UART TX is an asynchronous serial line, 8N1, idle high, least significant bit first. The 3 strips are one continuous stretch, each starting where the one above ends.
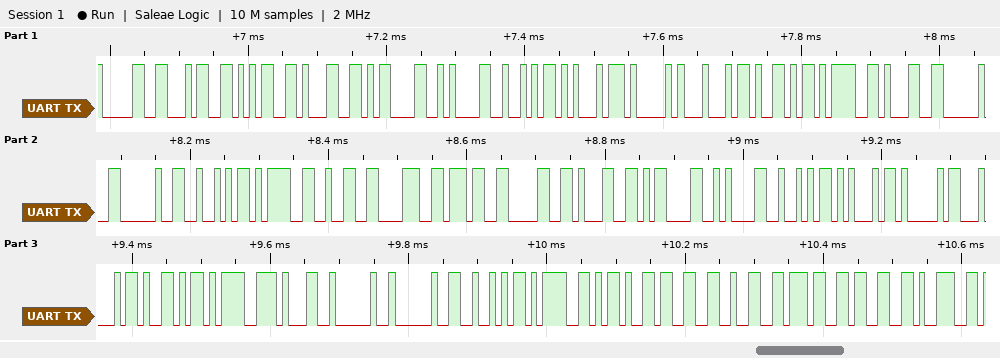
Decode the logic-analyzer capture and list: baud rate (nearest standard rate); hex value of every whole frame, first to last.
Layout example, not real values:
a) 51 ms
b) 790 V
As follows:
a) 115200 baud
b) 30 34 35 31 0D 0A 52 45 41 44 59 3D 31 20 20 52 3D 32 38 37 30 31 0D 0A 52 45 41 44 59 3D 31 20 20 52 3D 2D 33 32 37 33 39
